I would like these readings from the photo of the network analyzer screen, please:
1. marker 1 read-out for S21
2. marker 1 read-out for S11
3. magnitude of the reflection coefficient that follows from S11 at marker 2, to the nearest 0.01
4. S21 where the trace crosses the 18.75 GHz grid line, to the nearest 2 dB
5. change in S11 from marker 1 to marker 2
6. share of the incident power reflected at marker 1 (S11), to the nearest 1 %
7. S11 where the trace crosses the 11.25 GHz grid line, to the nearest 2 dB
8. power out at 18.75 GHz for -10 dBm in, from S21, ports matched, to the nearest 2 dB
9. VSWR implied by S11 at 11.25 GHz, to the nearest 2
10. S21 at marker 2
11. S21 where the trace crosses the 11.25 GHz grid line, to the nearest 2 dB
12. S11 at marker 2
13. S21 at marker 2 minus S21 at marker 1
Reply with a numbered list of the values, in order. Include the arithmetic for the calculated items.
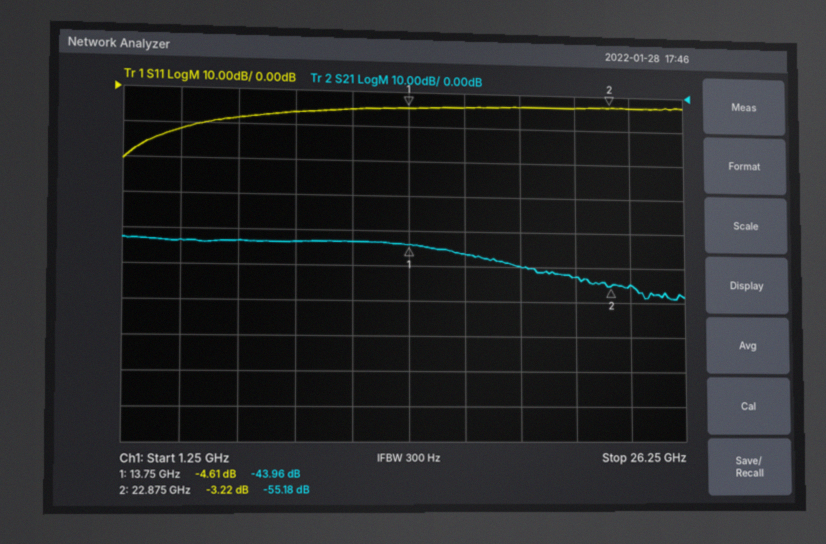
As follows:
1. -43.96 dB
2. -4.61 dB
3. 10^(-3.22/20) ≈ 0.69
4. -50 dB
5. -3.22 − (-4.61) = 1.39 dB
6. 10^(-4.61/10) ≈ 35 %
7. -6 dB
8. -10 dBm + (-50 dB) = -60 dBm
9. |Γ| = 10^(-6/20) = 0.5012; VSWR = (1 + 0.5012)/(1 − 0.5012) ≈ 3.01, so 4 to the nearest 2
10. -55.18 dB
11. -44 dB
12. -3.22 dB
13. -55.18 − (-43.96) = -11.22 dB
